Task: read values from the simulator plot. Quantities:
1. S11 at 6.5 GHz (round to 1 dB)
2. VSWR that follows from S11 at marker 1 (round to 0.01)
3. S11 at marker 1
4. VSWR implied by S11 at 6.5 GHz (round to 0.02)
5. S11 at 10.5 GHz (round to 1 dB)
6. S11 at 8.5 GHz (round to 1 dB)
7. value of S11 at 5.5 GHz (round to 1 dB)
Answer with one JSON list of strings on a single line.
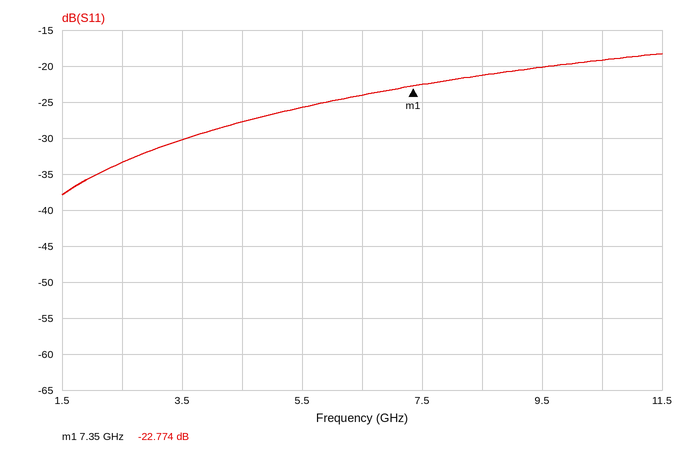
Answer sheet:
["-24 dB", "1.16", "-22.774 dB", "1.14", "-19 dB", "-21 dB", "-26 dB"]
